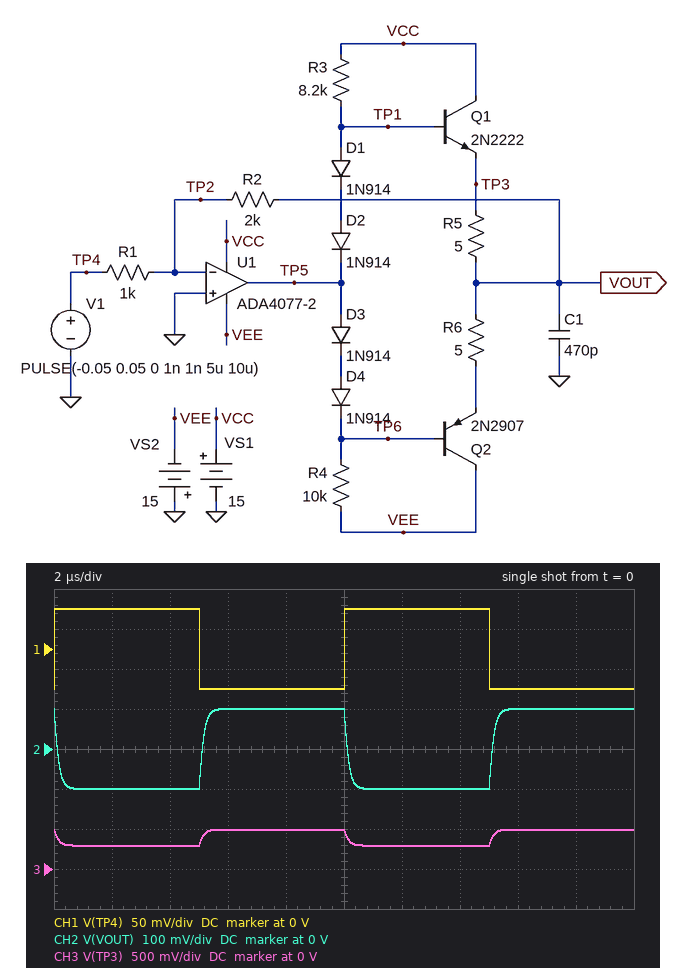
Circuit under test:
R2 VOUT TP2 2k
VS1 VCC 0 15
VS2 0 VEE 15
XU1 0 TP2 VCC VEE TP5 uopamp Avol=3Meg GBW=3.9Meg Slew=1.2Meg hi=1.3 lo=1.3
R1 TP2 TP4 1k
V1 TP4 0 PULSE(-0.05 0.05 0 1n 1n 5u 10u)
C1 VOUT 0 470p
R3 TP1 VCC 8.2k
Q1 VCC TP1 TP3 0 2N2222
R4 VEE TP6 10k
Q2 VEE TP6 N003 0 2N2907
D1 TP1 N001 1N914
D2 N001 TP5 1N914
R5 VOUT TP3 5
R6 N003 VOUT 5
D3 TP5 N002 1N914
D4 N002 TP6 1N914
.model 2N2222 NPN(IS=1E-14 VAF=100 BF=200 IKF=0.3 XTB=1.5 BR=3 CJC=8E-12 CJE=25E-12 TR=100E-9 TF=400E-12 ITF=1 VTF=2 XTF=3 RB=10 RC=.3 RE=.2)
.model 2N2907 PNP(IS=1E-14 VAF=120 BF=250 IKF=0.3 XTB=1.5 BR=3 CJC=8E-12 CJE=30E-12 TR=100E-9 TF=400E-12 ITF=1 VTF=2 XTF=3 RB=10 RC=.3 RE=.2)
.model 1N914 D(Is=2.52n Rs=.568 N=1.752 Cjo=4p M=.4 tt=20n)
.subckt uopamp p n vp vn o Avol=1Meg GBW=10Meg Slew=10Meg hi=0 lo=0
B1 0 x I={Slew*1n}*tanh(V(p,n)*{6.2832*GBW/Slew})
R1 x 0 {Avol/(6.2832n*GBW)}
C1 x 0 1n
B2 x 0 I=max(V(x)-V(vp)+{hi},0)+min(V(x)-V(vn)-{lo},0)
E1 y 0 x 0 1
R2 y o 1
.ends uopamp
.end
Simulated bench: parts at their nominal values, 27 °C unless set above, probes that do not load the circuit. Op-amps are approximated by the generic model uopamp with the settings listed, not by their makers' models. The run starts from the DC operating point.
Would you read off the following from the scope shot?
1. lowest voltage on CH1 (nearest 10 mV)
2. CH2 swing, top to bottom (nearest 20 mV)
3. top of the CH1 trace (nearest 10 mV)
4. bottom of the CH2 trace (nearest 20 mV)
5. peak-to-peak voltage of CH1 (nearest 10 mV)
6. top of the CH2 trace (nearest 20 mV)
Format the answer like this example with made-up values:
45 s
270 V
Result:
-50 mV
200 mV
50 mV
-100 mV
100 mV
100 mV
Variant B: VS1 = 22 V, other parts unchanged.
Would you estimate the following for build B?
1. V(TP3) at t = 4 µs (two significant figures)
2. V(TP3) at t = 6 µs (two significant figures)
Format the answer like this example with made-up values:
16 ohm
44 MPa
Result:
310 mV
510 mV
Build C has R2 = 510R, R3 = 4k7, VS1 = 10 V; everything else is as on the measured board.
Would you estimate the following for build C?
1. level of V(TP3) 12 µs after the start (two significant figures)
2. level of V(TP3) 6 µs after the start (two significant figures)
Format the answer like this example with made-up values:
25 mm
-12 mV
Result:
370 mV
420 mV
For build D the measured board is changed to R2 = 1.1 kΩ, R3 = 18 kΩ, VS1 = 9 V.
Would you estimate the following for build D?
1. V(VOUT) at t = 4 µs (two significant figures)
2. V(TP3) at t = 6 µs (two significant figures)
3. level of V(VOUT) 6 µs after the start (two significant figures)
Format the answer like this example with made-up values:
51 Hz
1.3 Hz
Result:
-55 mV
350 mV
55 mV
